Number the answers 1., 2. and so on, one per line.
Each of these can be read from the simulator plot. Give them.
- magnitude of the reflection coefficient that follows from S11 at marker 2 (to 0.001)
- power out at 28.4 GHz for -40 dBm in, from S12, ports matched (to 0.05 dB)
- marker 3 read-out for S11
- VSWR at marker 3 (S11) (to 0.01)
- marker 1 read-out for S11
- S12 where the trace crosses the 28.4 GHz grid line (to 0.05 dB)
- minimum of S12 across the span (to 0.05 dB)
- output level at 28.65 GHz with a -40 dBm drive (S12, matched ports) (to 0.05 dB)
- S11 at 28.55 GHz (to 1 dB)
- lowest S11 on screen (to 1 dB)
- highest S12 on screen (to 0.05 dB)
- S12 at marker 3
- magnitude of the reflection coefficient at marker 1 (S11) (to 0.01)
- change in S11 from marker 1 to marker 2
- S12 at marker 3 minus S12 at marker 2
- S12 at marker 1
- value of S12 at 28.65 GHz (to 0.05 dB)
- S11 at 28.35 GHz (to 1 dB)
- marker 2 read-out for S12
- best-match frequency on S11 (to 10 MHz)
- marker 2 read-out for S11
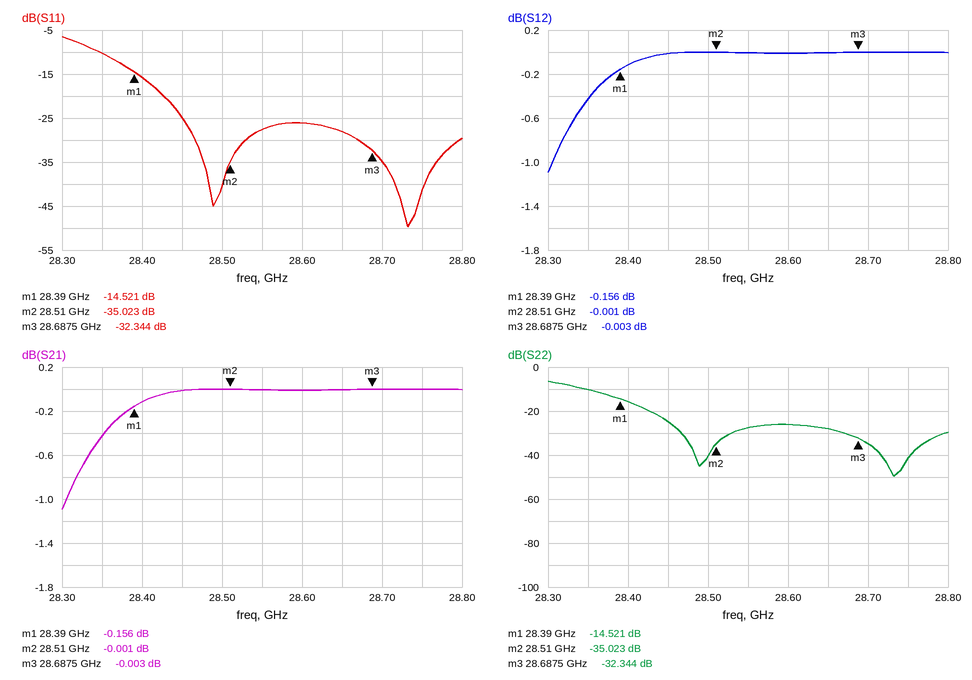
1. 0.018
2. -40.10 dBm
3. -32.344 dB
4. 1.05
5. -14.521 dB
6. -0.10 dB
7. -1.10 dB
8. -40.00 dBm
9. -28 dB
10. -50 dB
11. 0.00 dB
12. -0.003 dB
13. 0.19
14. -20.502 dB
15. -0.002 dB
16. -0.156 dB
17. 0.00 dB
18. -10 dB
19. -0.001 dB
20. 28.73 GHz
21. -35.023 dB
